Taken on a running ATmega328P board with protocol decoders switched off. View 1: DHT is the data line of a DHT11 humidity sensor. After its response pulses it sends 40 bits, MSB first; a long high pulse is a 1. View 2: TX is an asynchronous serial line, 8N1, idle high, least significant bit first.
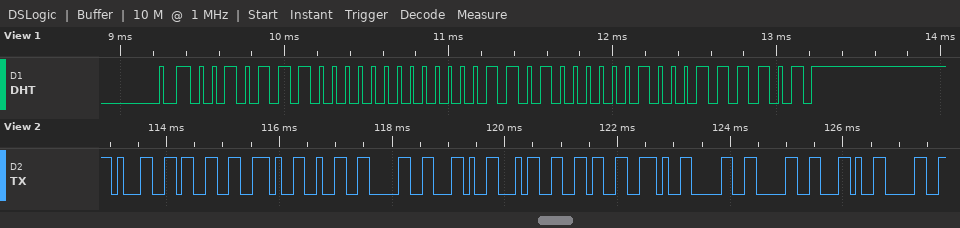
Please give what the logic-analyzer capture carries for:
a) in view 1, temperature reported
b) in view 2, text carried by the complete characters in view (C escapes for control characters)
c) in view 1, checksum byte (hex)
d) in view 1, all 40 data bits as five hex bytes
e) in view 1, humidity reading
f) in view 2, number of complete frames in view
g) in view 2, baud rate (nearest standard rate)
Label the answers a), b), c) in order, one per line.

a) 13.2 °C
b) "13.20,46.00,0"
c) 0x3D
d) 2E 00 0D 02 3D
e) 46 %
f) 13
g) 9600 baud
